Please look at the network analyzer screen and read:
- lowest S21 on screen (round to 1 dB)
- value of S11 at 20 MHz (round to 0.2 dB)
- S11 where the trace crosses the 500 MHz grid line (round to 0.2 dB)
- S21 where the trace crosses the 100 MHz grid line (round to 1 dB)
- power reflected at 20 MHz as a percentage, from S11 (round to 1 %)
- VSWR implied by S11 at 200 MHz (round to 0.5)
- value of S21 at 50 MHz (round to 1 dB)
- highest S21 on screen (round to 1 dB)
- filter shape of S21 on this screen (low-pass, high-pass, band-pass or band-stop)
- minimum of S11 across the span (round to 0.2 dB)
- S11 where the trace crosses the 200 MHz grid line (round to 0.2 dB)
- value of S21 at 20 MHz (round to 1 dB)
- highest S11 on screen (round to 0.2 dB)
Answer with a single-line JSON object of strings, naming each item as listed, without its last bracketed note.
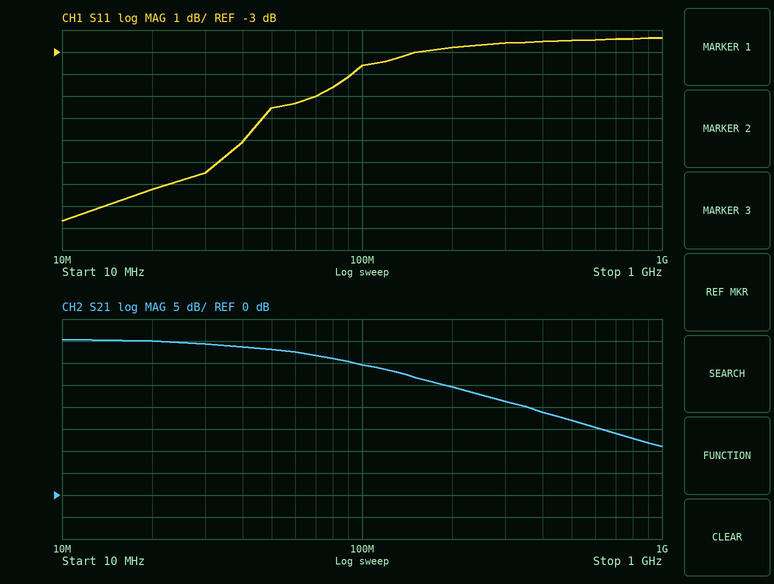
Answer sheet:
{"lowest S21 on screen": "11 dB", "value of S11 at 20 MHz": "-9.2 dB", "S11 where the trace crosses the 500 MHz grid line": "-2.4 dB", "S21 where the trace crosses the 100 MHz grid line": "30 dB", "power reflected at 20 MHz as a percentage, from S11": "12 %", "VSWR implied by S11 at 200 MHz": "6.5", "value of S21 at 50 MHz": "33 dB", "highest S21 on screen": "35 dB", "filter shape of S21 on this screen": "low-pass", "minimum of S11 across the span": "-10.6 dB", "S11 where the trace crosses the 200 MHz grid line": "-2.8 dB", "value of S21 at 20 MHz": "35 dB", "highest S11 on screen": "-2.4 dB"}
